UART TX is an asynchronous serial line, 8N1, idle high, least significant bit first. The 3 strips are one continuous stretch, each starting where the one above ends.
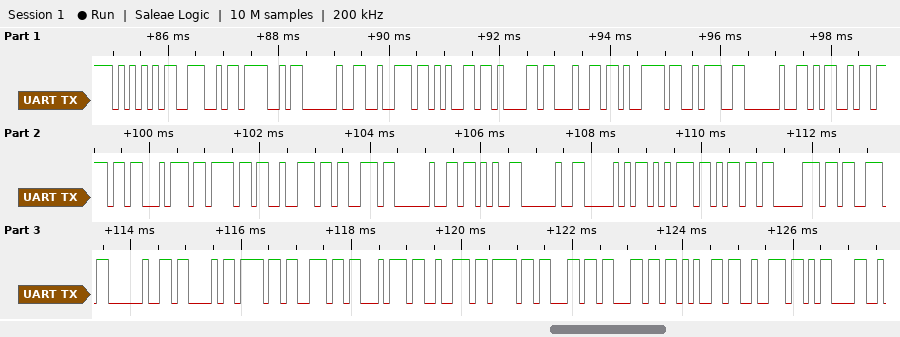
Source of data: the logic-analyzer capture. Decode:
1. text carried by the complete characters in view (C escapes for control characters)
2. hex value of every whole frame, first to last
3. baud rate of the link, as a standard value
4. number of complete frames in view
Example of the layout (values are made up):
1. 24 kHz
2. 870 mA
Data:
1. "UNO ready: Motors + Pumps Controller\r"
2. 55 4E 4F 20 72 65 61 64 79 3A 20 4D 6F 74 6F 72 73 20 2B 20 50 75 6D 70 73 20 43 6F 6E 74 72 6F 6C 6C 65 72 0D
3. 9600 baud
4. 37
